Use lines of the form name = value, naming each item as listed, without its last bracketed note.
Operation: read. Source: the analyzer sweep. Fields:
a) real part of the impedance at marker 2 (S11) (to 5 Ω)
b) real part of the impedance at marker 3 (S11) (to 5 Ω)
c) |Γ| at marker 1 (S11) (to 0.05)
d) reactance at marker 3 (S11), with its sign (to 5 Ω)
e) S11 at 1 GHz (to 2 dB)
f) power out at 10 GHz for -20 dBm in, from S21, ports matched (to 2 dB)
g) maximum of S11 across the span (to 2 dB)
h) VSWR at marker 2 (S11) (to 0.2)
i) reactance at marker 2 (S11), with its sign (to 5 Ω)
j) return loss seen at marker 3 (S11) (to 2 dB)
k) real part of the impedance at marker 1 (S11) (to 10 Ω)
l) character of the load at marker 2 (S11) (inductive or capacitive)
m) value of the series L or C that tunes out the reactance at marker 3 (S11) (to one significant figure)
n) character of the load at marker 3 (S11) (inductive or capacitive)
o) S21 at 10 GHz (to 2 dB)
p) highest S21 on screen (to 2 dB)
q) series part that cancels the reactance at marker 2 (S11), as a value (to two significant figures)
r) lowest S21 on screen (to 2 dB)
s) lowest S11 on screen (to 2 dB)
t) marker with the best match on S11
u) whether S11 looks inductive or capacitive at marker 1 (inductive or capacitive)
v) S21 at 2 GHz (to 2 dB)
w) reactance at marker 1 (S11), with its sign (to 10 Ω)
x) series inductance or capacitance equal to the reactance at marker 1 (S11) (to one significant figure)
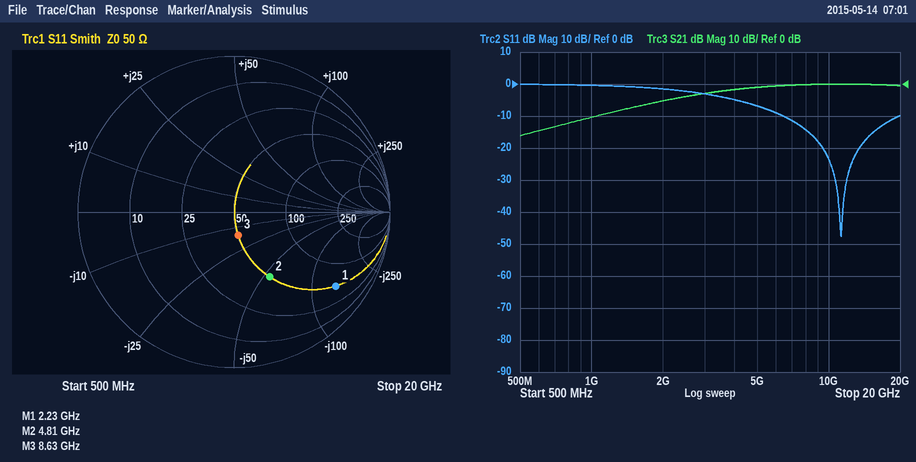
real part of the impedance at marker 2 (S11) = 50 Ω
real part of the impedance at marker 3 (S11) = 50 Ω
|Γ| at marker 1 (S11) = 0.80
reactance at marker 3 (S11), with its sign = -15 Ω
S11 at 1 GHz = 0 dB
power out at 10 GHz for -20 dBm in, from S21, ports matched = -20 dBm
maximum of S11 across the span = 0 dB
VSWR at marker 2 (S11) = 2.8
reactance at marker 2 (S11), with its sign = -55 Ω
return loss seen at marker 3 (S11) = 16 dB
real part of the impedance at marker 1 (S11) = 50 Ω
character of the load at marker 2 (S11) = capacitive
value of the series L or C that tunes out the reactance at marker 3 (S11) = 300 pH
character of the load at marker 3 (S11) = capacitive
S21 at 10 GHz = 0 dB
highest S21 on screen = 0 dB
series part that cancels the reactance at marker 2 (S11), as a value = 1.8 nH
lowest S21 on screen = -16 dB
lowest S11 on screen = -48 dB
marker with the best match on S11 = marker 3
whether S11 looks inductive or capacitive at marker 1 = capacitive
S21 at 2 GHz = -6 dB
reactance at marker 1 (S11), with its sign = -140 Ω
series inductance or capacitance equal to the reactance at marker 1 (S11) = 500 fF
